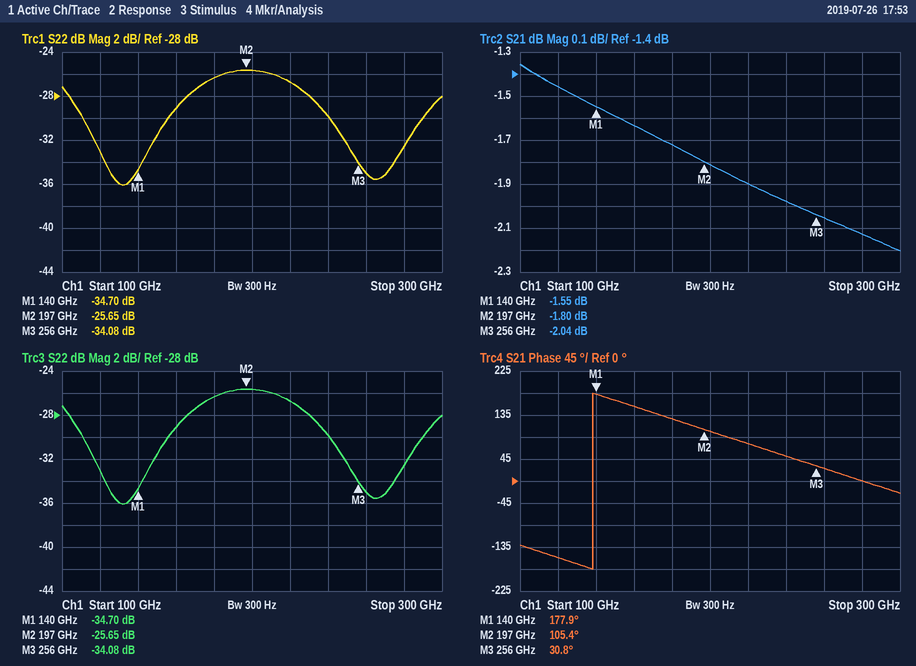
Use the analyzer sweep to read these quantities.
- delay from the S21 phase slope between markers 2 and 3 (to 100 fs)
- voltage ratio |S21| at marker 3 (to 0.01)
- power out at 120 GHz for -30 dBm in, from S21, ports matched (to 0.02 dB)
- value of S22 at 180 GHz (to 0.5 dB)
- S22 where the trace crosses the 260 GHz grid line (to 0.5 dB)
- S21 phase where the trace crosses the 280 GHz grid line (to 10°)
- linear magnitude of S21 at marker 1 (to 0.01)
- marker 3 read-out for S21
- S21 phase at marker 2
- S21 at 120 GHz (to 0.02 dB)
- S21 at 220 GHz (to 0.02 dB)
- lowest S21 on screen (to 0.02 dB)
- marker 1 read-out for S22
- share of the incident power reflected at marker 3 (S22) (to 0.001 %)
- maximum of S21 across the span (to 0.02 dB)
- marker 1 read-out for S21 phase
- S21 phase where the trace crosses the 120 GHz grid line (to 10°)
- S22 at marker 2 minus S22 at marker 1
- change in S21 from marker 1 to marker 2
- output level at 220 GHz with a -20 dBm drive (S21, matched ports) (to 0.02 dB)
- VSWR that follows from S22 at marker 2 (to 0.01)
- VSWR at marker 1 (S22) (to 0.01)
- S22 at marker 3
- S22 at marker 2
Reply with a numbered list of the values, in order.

1. 3.5 ps
2. 0.79
3. -31.46 dBm
4. -26.5 dB
5. -35.0 dB
6. 0°
7. 0.84
8. -2.04 dB
9. 105.4°
10. -1.46 dB
11. -1.90 dB
12. -2.20 dB
13. -34.70 dB
14. 0.039 %
15. -1.36 dB
16. 177.9°
17. -160°
18. 9.05 dB
19. -0.25 dB
20. -21.90 dBm
21. 1.11
22. 1.04
23. -34.08 dB
24. -25.65 dB
